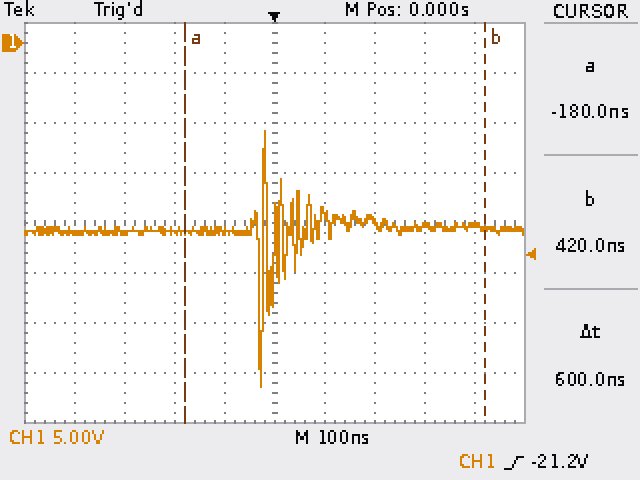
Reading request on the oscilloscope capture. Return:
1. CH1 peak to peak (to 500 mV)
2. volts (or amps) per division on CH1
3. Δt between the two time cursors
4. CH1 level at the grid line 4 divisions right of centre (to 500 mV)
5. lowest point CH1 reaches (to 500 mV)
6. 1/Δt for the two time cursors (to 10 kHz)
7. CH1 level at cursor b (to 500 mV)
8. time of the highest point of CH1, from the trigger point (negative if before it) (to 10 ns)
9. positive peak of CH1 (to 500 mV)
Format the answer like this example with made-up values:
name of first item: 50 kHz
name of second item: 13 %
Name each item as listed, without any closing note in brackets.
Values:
CH1 peak to peak: 25.5 V
volts (or amps) per division on CH1: 5 V
Δt between the two time cursors: 600 ns
CH1 level at the grid line 4 divisions right of centre: -18.0 V
lowest point CH1 reaches: -34.5 V
1/Δt for the two time cursors: 1.67 MHz
CH1 level at cursor b: -18.5 V
time of the highest point of CH1, from the trigger point (negative if before it): -20 ns
positive peak of CH1: -9.0 V
